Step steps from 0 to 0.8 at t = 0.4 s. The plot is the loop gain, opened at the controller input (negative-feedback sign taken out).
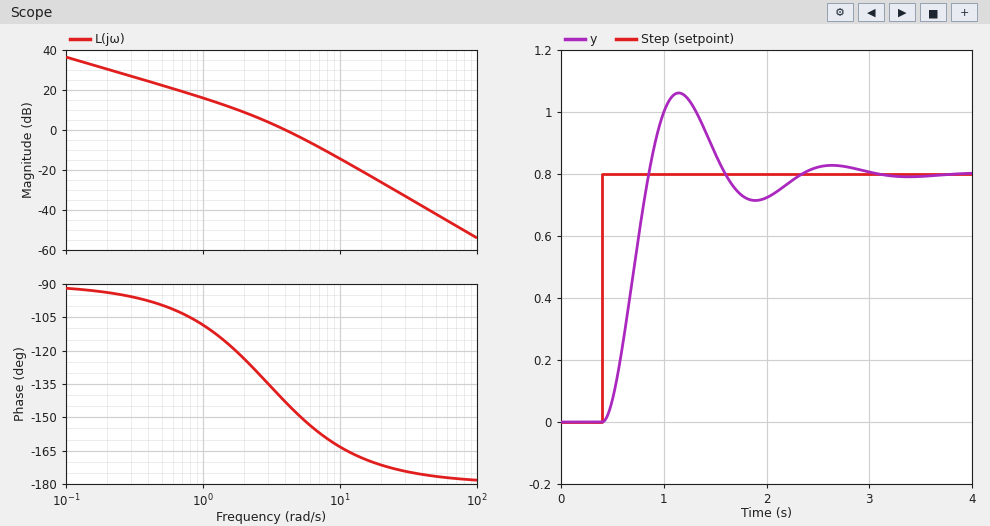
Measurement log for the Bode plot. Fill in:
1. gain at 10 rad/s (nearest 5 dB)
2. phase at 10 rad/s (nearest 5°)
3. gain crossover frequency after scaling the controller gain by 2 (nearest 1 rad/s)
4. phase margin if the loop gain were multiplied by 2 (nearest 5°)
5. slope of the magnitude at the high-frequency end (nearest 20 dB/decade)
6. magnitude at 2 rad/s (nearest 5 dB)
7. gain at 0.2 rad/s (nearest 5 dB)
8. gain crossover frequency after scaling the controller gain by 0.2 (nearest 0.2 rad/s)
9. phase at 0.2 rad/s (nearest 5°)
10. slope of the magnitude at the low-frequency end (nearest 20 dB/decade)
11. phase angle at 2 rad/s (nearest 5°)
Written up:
-15 dB
-165°
6 rad/s
25°
-40 dB/decade
10 dB
30 dB
1.2 rad/s
-95°
-20 dB/decade
-125°
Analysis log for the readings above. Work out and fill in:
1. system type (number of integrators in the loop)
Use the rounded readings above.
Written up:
1
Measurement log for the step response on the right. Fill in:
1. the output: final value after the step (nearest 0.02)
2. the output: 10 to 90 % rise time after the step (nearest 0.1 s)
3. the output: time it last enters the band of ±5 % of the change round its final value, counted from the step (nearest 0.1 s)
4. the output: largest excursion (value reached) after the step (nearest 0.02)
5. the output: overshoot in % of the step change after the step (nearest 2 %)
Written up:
0.80
0.3 s
1.8 s
1.06
32 %
